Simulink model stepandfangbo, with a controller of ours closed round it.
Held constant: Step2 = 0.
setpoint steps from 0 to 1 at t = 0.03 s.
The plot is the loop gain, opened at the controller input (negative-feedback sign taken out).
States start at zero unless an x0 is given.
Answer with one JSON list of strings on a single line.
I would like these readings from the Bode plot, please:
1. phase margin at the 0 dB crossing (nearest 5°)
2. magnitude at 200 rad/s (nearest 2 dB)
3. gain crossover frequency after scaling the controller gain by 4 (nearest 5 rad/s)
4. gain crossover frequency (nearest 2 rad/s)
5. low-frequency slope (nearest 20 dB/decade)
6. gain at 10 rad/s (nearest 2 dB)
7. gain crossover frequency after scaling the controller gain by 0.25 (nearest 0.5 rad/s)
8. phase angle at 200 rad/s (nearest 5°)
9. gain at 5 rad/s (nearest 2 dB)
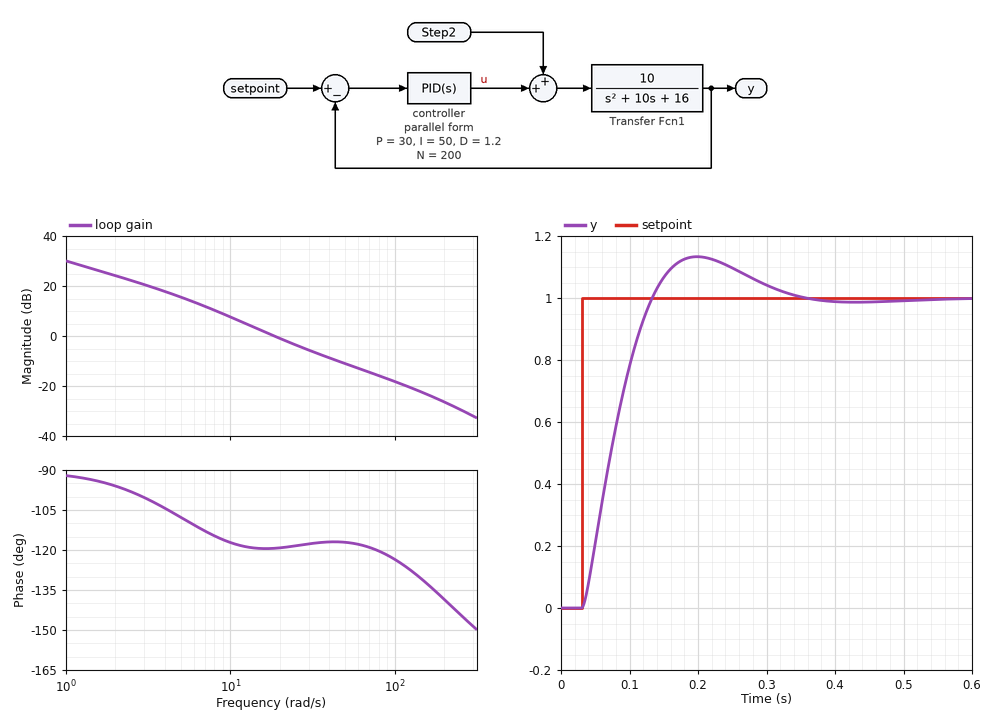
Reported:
["60°", "-26 dB", "55 rad/s", "18 rad/s", "-20 dB/decade", "8 dB", "7.0 rad/s", "-140°", "16 dB"]
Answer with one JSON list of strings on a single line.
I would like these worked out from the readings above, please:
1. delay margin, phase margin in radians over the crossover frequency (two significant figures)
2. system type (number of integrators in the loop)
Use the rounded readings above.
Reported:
["0.058 s", "1"]
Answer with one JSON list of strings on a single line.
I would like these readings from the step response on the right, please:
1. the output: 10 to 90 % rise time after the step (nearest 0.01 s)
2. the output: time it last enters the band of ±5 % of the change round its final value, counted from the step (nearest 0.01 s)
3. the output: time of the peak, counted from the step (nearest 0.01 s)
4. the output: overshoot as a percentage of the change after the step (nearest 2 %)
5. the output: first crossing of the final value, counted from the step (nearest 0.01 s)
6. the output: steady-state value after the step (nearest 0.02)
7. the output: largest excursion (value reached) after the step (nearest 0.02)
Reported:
["0.07 s", "0.26 s", "0.17 s", "14 %", "0.10 s", "1.00", "1.14"]
